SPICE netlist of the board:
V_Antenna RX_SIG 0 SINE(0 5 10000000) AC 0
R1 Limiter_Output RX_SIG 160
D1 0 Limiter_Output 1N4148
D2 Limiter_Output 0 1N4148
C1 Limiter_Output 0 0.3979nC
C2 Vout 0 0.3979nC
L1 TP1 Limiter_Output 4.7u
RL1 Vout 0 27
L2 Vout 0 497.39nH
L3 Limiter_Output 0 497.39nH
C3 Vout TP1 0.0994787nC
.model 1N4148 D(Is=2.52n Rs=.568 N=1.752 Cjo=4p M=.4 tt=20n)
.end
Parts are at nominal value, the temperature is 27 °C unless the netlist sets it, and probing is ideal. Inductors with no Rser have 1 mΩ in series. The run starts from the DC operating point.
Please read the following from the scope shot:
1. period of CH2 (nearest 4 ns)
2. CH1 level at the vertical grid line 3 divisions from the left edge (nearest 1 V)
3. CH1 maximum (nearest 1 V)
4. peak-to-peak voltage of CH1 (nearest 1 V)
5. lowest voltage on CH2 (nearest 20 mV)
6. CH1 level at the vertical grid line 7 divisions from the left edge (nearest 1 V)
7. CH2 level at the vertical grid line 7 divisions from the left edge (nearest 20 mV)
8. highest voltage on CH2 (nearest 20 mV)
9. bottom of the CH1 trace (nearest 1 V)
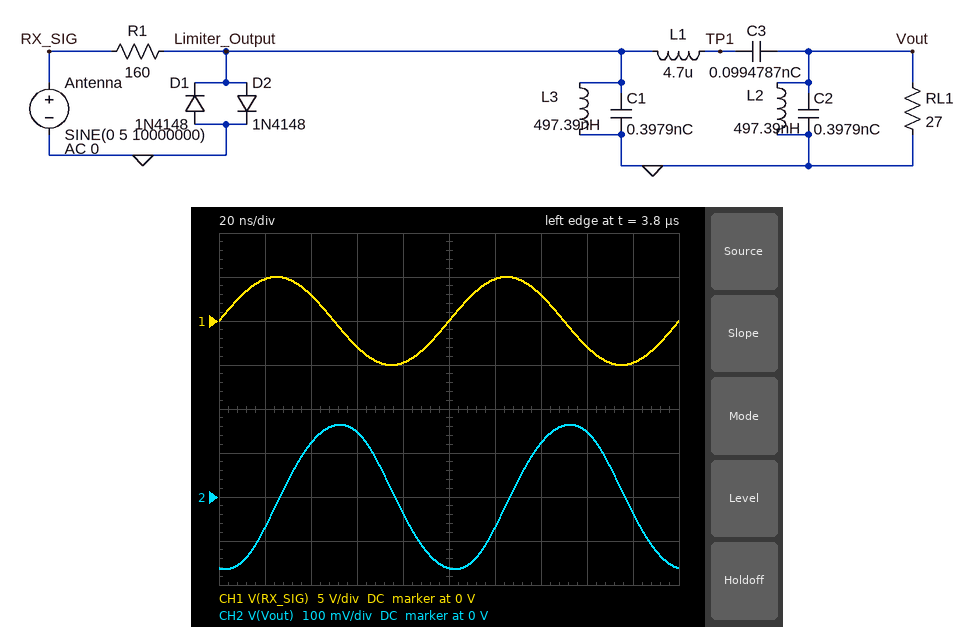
100 ns
-3 V
5 V
10 V
-160 mV
3 V
120 mV
160 mV
-5 V
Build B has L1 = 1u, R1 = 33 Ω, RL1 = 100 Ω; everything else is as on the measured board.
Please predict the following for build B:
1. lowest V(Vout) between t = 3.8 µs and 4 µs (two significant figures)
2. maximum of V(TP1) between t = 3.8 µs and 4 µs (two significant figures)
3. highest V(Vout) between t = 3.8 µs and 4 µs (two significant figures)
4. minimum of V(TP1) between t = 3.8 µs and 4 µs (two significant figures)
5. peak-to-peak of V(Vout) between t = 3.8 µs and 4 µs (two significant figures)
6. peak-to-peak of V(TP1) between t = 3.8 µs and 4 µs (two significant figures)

-960 mV
1.7 V
960 mV
-1.7 V
1.9 V
3.4 V
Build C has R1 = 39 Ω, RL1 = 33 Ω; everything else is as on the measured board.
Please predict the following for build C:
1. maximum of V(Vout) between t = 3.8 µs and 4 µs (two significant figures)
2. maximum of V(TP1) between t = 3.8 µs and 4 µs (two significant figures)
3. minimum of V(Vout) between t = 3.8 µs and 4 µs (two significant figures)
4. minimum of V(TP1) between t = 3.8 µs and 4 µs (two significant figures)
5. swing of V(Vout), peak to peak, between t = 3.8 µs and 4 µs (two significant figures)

220 mV
1.1 V
-220 mV
-1.1 V
440 mV
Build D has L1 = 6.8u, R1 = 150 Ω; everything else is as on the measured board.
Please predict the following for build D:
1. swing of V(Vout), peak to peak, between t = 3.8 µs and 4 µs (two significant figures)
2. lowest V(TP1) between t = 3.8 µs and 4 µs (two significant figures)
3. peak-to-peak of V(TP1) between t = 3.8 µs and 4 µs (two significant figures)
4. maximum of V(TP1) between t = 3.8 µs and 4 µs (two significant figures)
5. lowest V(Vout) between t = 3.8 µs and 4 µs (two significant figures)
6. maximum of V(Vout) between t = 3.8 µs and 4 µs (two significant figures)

170 mV
-510 mV
1.0 V
510 mV
-86 mV
86 mV
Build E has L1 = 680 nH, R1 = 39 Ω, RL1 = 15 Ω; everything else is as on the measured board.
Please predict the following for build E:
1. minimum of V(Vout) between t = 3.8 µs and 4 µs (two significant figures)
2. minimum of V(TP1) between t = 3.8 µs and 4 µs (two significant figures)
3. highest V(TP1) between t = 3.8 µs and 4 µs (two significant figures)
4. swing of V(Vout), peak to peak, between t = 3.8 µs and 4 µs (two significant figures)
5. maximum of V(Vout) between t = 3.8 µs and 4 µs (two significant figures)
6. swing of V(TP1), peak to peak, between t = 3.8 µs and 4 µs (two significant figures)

-140 mV
-1.6 V
1.6 V
290 mV
140 mV
3.2 V
